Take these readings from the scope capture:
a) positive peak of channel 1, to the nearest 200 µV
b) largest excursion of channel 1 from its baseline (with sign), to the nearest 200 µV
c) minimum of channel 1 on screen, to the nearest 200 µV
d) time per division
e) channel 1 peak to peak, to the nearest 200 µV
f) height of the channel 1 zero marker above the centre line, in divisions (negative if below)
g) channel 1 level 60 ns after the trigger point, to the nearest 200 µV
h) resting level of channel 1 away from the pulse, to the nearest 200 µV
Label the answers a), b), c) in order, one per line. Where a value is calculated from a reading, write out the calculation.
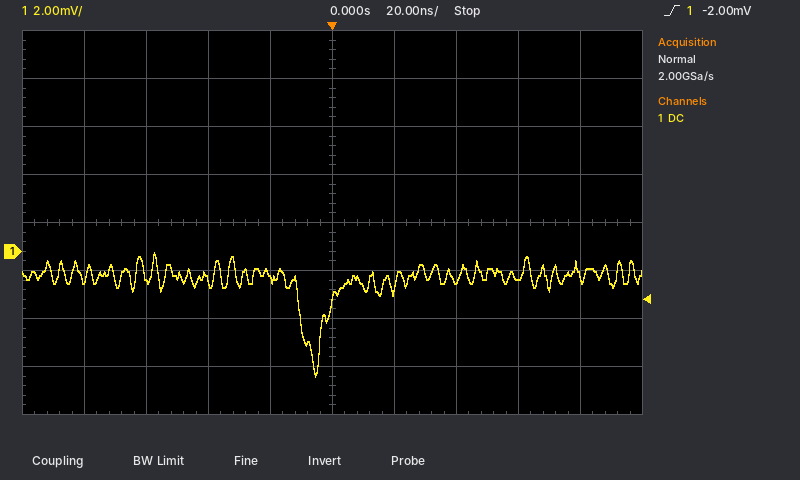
a) 0.0 mV
b) -5.2 mV − (-1.0 mV) = -4.2 mV
c) -5.2 mV
d) 20 ns
e) 0.0 mV − (-5.2 mV) = 5.2 mV
f) -0.6 div
g) -1.2 mV
h) -1.0 mV
